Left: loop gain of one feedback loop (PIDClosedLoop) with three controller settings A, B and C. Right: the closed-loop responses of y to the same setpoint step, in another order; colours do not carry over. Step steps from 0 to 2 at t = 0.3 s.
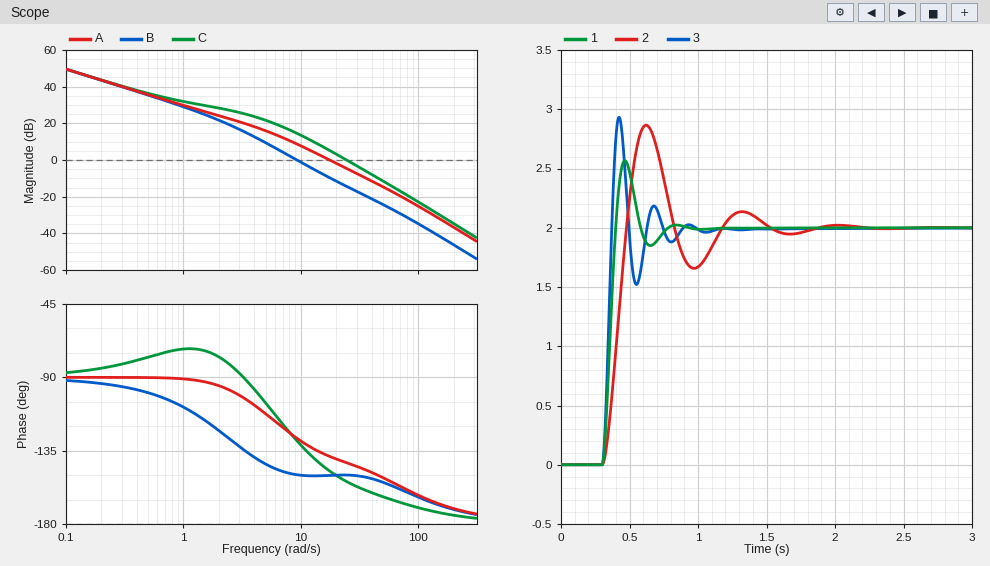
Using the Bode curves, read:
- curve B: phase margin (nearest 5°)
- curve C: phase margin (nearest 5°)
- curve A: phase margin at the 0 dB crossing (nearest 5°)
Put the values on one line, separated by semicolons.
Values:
30°; 25°; 40°
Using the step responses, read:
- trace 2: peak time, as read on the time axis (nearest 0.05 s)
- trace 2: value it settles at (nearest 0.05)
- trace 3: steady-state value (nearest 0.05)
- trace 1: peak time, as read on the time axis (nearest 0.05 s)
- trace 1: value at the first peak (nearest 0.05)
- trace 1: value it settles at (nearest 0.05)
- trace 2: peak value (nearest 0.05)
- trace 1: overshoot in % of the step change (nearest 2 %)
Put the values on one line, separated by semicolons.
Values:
0.60 s; 2.00; 2.00; 0.45 s; 2.55; 2.00; 2.85; 28 %
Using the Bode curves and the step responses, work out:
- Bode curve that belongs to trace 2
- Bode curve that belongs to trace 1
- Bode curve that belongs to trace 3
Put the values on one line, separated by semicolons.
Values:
B; A; C
